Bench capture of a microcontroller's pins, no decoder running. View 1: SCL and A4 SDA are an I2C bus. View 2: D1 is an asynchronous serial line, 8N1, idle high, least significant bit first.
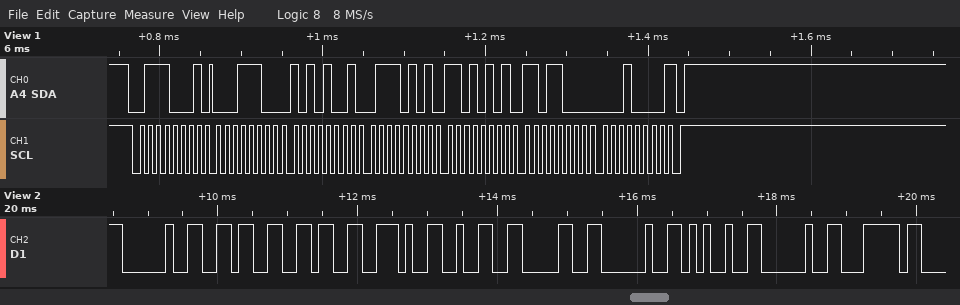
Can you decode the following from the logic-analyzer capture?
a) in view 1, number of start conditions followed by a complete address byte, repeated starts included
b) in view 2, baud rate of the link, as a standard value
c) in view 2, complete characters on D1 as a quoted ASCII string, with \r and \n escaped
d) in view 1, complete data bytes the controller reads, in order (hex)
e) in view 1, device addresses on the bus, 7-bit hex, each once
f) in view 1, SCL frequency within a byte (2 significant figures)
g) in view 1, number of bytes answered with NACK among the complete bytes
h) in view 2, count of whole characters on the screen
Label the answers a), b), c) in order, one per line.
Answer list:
a) 1
b) 9600 baud
c) " 66.20 % |"
d) 1C A9 75 D5 D8 10
e) 0x38
f) 100 kHz
g) 1
h) 10
